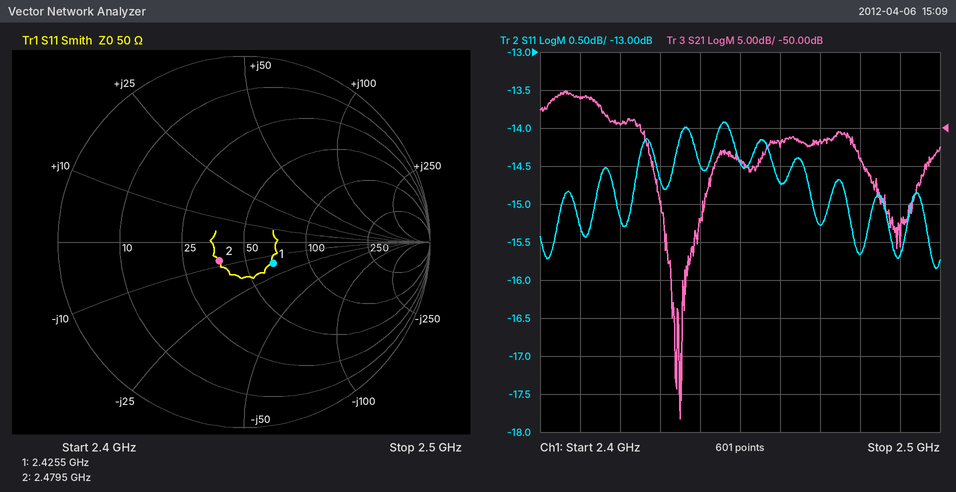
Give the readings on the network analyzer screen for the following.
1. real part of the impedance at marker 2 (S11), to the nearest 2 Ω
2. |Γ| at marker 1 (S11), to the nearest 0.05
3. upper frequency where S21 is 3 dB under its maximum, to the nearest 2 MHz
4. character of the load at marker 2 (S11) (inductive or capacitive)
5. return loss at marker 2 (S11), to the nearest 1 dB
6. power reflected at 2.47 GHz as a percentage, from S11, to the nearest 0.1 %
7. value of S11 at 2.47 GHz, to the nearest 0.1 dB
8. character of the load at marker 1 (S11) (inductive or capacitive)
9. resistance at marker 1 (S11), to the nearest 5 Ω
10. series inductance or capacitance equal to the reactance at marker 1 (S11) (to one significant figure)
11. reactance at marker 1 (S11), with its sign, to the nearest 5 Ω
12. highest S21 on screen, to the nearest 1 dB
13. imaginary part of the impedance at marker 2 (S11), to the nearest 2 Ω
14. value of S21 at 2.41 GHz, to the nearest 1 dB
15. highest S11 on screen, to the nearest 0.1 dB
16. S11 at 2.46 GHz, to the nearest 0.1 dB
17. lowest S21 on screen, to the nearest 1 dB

38 Ω
0.20
2.416 GHz
capacitive
16 dB
3.0 %
-15.3 dB
capacitive
65 Ω
4 pF
-15 Ω
-45 dB
-8 Ω
-46 dB
-13.9 dB
-14.7 dB
-88 dB
